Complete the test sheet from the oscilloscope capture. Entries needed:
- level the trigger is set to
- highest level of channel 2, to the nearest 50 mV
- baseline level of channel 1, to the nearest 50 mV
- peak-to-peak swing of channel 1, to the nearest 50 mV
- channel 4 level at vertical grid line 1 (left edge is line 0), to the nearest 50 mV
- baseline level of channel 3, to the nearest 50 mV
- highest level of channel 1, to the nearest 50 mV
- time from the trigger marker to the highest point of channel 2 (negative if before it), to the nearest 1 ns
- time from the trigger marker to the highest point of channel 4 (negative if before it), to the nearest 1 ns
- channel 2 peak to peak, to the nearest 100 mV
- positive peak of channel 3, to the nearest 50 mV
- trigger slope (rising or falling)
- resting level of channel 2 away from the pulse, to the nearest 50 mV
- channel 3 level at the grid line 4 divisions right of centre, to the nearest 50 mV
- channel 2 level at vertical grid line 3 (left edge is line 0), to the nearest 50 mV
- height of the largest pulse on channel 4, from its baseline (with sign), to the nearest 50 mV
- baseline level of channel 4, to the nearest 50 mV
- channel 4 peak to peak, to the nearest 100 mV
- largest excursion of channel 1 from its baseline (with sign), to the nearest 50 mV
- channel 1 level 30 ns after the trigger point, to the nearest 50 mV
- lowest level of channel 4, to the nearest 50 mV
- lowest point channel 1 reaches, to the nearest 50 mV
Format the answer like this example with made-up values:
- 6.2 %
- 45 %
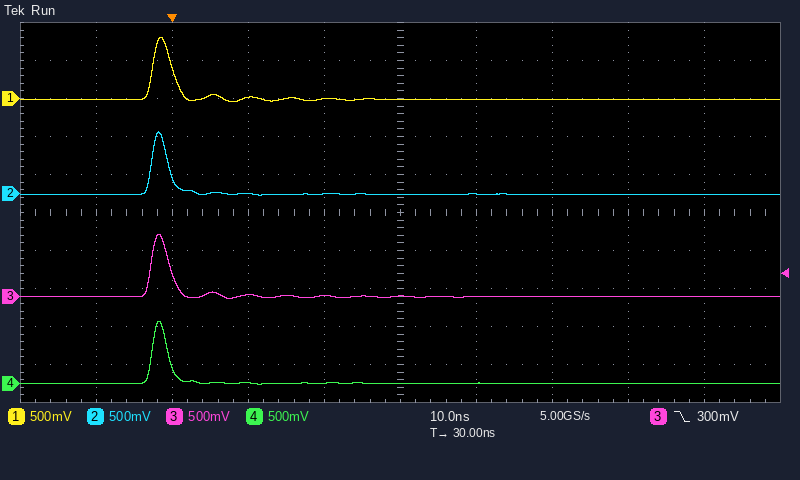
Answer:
- 300 mV
- 800 mV
- 0 mV
- 850 mV
- 0 mV
- 0 mV
- 800 mV
- -2 ns
- -2 ns
- 800 mV
- 800 mV
- falling
- 0 mV
- 0 mV
- 0 mV
- +800 mV
- 0 mV
- 800 mV
- +800 mV
- 0 mV
- 0 mV
- -50 mV
